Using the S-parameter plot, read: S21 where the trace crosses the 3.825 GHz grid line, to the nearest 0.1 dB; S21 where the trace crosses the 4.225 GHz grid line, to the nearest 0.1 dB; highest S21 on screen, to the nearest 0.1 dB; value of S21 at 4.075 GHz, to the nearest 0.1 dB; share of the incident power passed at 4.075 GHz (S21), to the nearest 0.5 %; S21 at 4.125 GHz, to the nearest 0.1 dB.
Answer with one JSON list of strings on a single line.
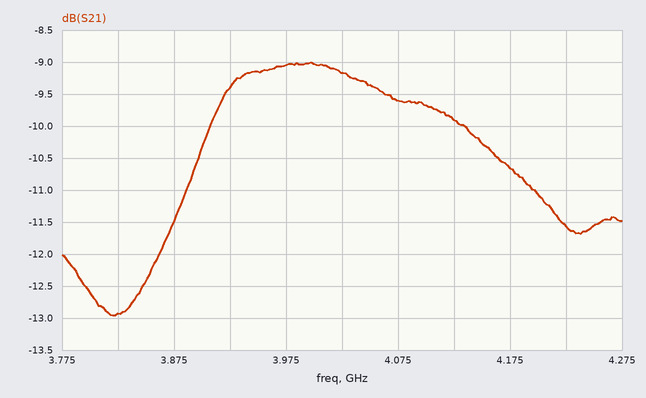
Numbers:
["-12.9 dB", "-11.6 dB", "-9.0 dB", "-9.6 dB", "11.0 %", "-9.9 dB"]
